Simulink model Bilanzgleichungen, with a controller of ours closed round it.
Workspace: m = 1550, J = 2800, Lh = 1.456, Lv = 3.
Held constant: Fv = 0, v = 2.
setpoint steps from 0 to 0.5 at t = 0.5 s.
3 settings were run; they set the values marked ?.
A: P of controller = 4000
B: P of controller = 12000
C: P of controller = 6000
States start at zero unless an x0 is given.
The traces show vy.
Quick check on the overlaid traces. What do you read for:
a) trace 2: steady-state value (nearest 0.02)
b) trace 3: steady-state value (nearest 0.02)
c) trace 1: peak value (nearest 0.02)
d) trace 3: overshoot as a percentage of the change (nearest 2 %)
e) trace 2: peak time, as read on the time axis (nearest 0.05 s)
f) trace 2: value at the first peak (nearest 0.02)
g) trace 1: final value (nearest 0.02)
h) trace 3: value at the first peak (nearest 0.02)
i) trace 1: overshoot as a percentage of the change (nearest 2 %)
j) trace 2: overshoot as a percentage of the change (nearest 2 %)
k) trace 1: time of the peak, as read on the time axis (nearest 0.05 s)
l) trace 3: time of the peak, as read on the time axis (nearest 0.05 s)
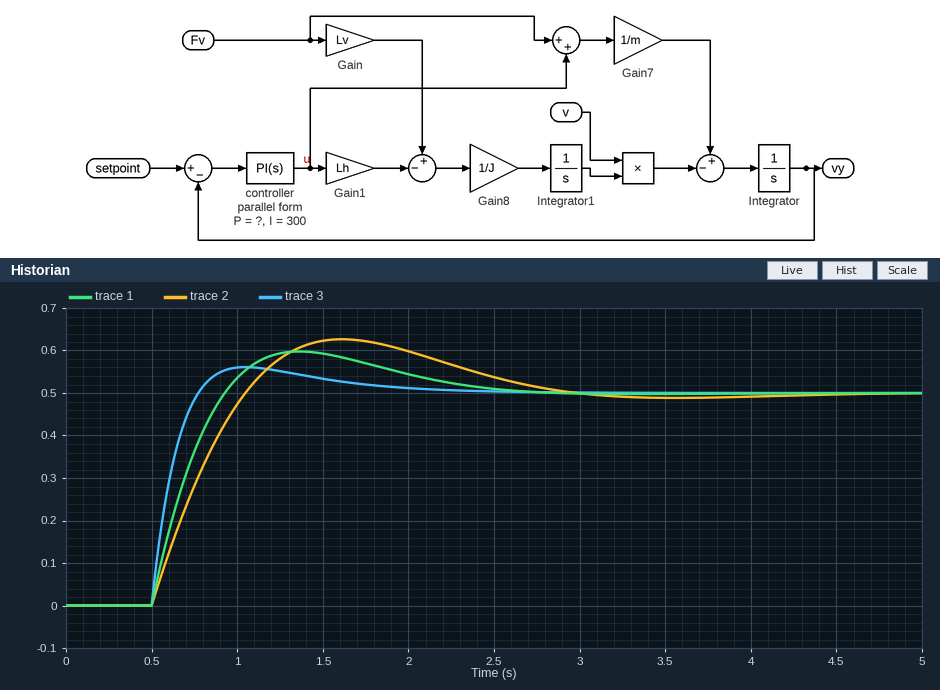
0.50
0.50
0.60
12 %
1.60 s
0.62
0.50
0.56
20 %
26 %
1.35 s
1.05 s
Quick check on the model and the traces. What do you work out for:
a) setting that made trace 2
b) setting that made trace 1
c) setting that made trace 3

A
C
B
